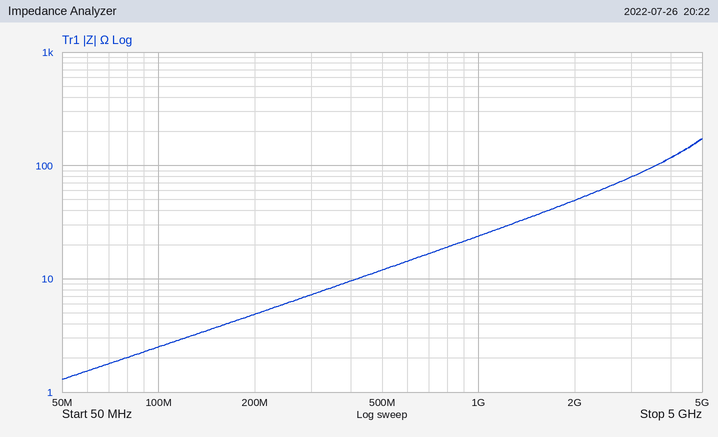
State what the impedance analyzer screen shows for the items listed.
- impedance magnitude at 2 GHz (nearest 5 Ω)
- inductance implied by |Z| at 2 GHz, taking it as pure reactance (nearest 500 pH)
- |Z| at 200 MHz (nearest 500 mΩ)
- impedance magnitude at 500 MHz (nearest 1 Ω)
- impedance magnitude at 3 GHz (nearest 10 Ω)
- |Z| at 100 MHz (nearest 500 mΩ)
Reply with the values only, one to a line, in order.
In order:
50 Ω
4.0 nH
5.0 Ω
12 Ω
80 Ω
2.5 Ω
